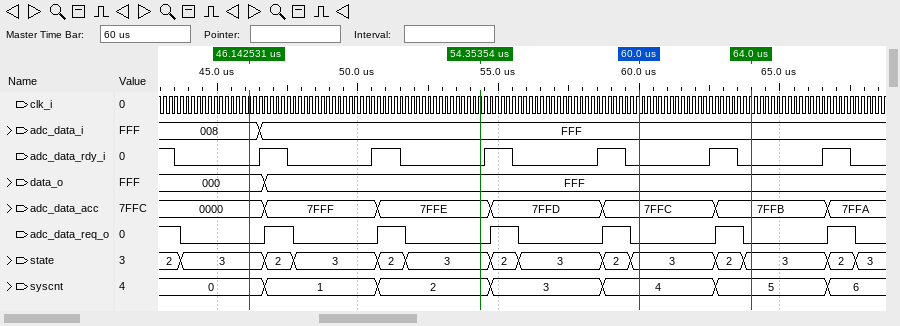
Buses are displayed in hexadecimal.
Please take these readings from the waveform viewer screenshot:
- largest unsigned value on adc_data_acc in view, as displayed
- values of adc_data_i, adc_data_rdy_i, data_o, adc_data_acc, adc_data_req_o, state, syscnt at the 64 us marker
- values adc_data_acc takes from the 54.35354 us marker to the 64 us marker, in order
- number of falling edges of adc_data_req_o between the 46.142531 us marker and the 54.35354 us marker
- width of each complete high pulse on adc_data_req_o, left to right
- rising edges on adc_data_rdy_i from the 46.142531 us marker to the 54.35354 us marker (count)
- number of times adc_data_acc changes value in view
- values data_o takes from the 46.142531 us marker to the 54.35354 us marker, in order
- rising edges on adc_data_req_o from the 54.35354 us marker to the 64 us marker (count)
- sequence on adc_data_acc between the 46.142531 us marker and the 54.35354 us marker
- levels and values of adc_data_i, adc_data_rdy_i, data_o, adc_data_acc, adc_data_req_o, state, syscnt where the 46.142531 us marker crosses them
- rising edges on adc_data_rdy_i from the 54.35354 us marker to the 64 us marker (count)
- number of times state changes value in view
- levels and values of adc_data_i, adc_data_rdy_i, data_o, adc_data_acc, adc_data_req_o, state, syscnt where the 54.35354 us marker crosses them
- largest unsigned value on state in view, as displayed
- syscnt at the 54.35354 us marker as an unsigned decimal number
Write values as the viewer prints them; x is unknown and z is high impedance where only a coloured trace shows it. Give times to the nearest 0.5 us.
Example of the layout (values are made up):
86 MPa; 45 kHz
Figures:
7FFF; adc_data_i=FFF, adc_data_rdy_i=0, data_o=FFF, adc_data_acc=7FFB, adc_data_req_o=0, state=3, syscnt=5; 7FFE, 7FFD, 7FFC, 7FFB; 2; 1 us, 1 us, 1 us, 1 us, 1 us, 1 us; 2; 6; 000, FFF; 3; 0000, 7FFF, 7FFE; adc_data_i=008, adc_data_rdy_i=0, data_o=000, adc_data_acc=0000, adc_data_req_o=0, state=3, syscnt=0; 3; 13; adc_data_i=FFF, adc_data_rdy_i=0, data_o=FFF, adc_data_acc=7FFE, adc_data_req_o=0, state=3, syscnt=2; 3; 2
